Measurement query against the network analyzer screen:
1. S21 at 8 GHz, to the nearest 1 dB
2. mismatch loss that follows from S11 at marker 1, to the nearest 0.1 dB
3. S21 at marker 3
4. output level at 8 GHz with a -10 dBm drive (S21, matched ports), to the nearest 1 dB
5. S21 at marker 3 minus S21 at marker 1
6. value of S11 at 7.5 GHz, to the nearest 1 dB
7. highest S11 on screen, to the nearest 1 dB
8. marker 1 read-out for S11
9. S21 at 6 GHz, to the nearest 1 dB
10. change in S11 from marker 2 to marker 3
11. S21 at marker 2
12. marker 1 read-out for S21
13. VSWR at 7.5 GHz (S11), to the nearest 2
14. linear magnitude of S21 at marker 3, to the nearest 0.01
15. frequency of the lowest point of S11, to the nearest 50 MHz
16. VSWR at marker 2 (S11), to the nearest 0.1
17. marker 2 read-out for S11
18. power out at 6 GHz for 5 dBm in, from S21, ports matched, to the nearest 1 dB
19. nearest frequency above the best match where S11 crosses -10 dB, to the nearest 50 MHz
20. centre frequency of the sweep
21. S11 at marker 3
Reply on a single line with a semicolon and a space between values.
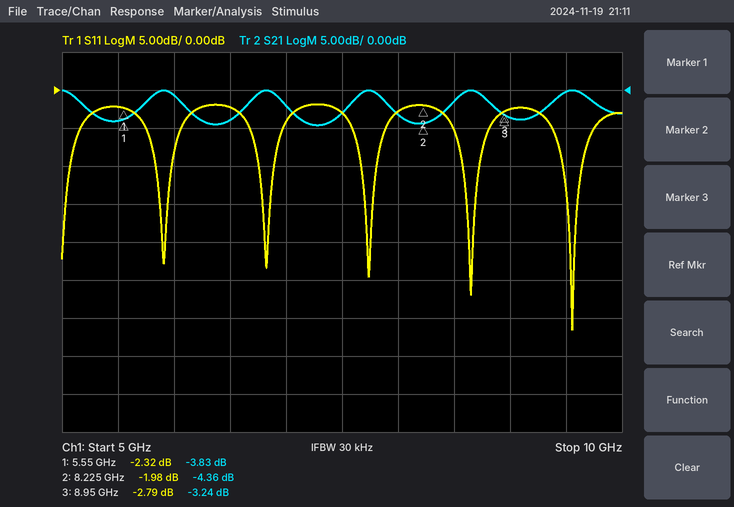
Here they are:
-3 dB; 3.8 dB; -3.24 dB; -13 dBm; 0.59 dB; -3 dB; -2 dB; -2.32 dB; -1 dB; -0.81 dB; -4.36 dB; -3.83 dB; 6; 0.69; 9.55 GHz; 8.8; -1.98 dB; 4 dBm; 9.65 GHz; 7.5 GHz; -2.79 dB
